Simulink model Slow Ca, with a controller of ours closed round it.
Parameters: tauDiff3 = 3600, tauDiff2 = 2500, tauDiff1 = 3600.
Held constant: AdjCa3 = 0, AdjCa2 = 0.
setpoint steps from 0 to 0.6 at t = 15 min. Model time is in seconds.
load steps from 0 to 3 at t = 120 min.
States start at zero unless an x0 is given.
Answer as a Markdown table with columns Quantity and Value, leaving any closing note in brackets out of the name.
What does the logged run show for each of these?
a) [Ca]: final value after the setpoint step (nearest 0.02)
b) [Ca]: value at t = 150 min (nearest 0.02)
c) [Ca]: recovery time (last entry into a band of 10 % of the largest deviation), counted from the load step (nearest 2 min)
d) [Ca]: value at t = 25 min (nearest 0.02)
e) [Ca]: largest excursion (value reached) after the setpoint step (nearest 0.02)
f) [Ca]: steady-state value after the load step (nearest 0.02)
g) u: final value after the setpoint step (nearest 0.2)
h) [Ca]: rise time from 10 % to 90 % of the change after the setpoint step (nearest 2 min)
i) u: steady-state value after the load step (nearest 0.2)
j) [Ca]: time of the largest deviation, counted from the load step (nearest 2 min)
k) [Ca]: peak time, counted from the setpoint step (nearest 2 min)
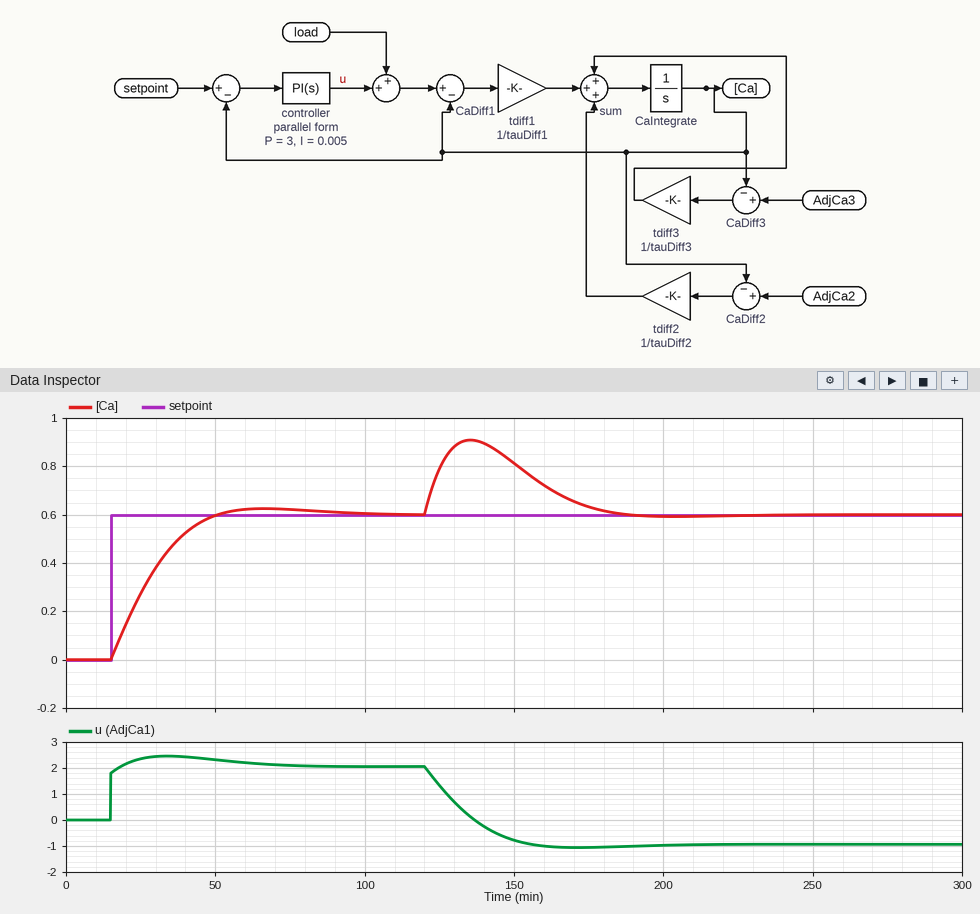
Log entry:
| Quantity | Value |
|---|---|
| [Ca]: final value after the setpoint step | 0.60 |
| [Ca]: value at t = 150 min | 0.82 |
| [Ca]: recovery time (last entry into a band of 10 % of the largest deviation), counted from the load step | 56 min |
| [Ca]: value at t = 25 min | 0.28 |
| [Ca]: largest excursion (value reached) after the setpoint step | 0.62 |
| [Ca]: steady-state value after the load step | 0.60 |
| u: final value after the setpoint step | 2.0 |
| [Ca]: rise time from 10 % to 90 % of the change after the setpoint step | 24 min |
| u: steady-state value after the load step | -1.0 |
| [Ca]: time of the largest deviation, counted from the load step | 16 min |
| [Ca]: peak time, counted from the setpoint step | 52 min |
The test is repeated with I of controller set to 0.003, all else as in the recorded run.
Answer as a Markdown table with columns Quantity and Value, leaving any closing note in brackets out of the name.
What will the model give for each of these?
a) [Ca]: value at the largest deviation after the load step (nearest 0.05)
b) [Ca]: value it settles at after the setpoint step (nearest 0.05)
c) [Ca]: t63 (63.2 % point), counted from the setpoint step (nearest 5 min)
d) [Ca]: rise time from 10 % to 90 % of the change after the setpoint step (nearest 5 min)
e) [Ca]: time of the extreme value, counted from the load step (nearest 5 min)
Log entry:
| Quantity | Value |
|---|---|
| [Ca]: value at the largest deviation after the load step | 0.95 |
| [Ca]: value it settles at after the setpoint step | 0.60 |
| [Ca]: t63 (63.2 % point), counted from the setpoint step | 20 min |
| [Ca]: rise time from 10 % to 90 % of the change after the setpoint step | 40 min |
| [Ca]: time of the extreme value, counted from the load step | 20 min |
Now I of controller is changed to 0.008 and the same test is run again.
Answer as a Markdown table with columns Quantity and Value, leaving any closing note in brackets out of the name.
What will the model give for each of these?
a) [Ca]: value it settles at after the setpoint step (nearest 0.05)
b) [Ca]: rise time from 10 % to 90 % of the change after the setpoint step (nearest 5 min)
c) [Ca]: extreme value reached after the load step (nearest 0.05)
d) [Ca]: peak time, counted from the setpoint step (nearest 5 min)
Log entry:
| Quantity | Value |
|---|---|
| [Ca]: value it settles at after the setpoint step | 0.60 |
| [Ca]: rise time from 10 % to 90 % of the change after the setpoint step | 15 min |
| [Ca]: extreme value reached after the load step | 0.90 |
| [Ca]: peak time, counted from the setpoint step | 35 min |
